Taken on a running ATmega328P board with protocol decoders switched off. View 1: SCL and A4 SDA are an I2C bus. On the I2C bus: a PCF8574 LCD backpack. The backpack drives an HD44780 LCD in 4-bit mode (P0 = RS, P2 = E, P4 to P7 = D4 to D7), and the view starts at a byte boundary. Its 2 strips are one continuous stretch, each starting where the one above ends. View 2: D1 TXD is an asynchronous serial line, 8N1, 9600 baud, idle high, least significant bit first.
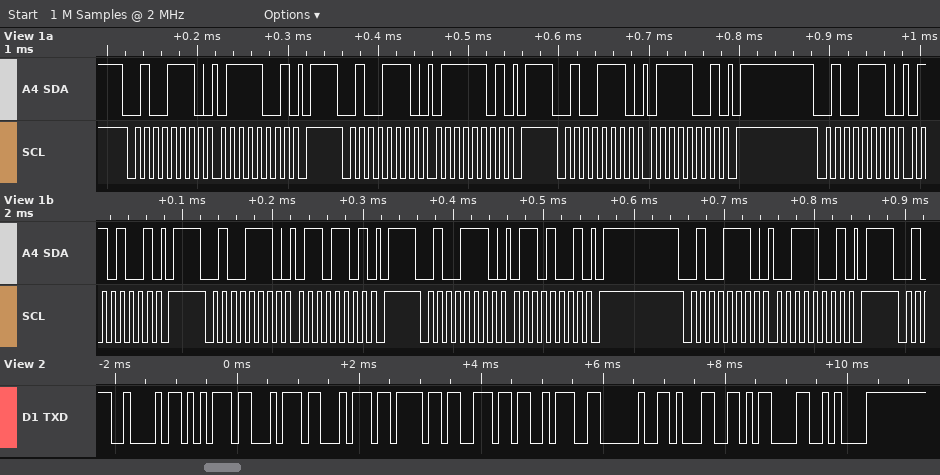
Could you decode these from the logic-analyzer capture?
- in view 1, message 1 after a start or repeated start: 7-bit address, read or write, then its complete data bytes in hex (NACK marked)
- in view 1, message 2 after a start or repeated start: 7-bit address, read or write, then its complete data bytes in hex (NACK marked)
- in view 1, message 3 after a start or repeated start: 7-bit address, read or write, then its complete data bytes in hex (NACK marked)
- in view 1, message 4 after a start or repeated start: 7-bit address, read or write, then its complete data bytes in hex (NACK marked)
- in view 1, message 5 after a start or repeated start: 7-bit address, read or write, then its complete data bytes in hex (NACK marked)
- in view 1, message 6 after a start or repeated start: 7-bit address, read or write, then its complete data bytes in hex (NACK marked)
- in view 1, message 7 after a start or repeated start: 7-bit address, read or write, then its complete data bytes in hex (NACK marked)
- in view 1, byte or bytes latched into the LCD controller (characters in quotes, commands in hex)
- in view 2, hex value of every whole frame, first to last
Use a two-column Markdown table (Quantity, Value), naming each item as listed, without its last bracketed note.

| Quantity | Value |
|---|---|
| in view 1, message 1 after a start or repeated start: 7-bit address, read or write, then its complete data bytes in hex | 0x27 write: 79 |
| in view 1, message 2 after a start or repeated start: 7-bit address, read or write, then its complete data bytes in hex | 0x27 write: 7D |
| in view 1, message 3 after a start or repeated start: 7-bit address, read or write, then its complete data bytes in hex | 0x27 write: 79 |
| in view 1, message 4 after a start or repeated start: 7-bit address, read or write, then its complete data bytes in hex | 0x27 write: 69 |
| in view 1, message 5 after a start or repeated start: 7-bit address, read or write, then its complete data bytes in hex | 0x27 write: 6D |
| in view 1, message 6 after a start or repeated start: 7-bit address, read or write, then its complete data bytes in hex | 0x27 write: 69 |
| in view 1, message 7 after a start or repeated start: 7-bit address, read or write, then its complete data bytes in hex | 0x27 write: 39 |
| in view 1, byte or bytes latched into the LCD controller | 'v' |
| in view 2, hex value of every whole frame, first to last | 42 75 74 74 6F 6E 3A 20 31 0D 0A |
